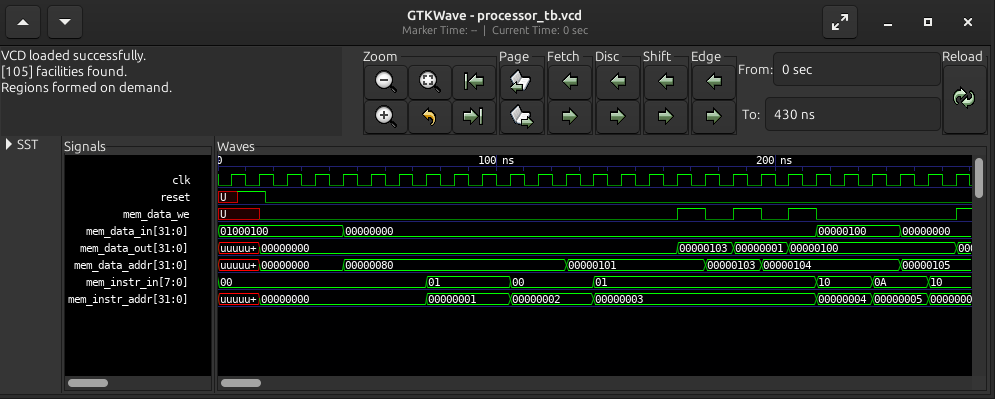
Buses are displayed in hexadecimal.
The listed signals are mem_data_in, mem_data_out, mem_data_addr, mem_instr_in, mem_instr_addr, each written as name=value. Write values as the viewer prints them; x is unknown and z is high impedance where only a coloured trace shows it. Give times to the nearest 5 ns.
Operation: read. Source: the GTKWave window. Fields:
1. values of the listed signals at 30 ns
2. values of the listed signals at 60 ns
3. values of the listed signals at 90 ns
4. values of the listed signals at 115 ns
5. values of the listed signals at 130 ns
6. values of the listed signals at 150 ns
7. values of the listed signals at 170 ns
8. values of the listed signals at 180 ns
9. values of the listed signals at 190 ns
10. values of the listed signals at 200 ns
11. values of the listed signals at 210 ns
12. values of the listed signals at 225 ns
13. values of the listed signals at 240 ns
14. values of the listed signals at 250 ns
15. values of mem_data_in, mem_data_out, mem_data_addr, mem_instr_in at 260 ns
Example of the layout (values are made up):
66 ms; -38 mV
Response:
mem_data_in=01000100, mem_data_out=00000000, mem_data_addr=00000000, mem_instr_in=00, mem_instr_addr=00000000; mem_data_in=00000000, mem_data_out=00000000, mem_data_addr=00000080, mem_instr_in=00, mem_instr_addr=00000000; mem_data_in=00000000, mem_data_out=00000000, mem_data_addr=00000080, mem_instr_in=01, mem_instr_addr=00000001; mem_data_in=00000000, mem_data_out=00000000, mem_data_addr=00000080, mem_instr_in=00, mem_instr_addr=00000002; mem_data_in=00000000, mem_data_out=00000000, mem_data_addr=00000101, mem_instr_in=00, mem_instr_addr=00000002; mem_data_in=00000000, mem_data_out=00000000, mem_data_addr=00000101, mem_instr_in=01, mem_instr_addr=00000003; mem_data_in=00000000, mem_data_out=00000103, mem_data_addr=00000101, mem_instr_in=01, mem_instr_addr=00000003; mem_data_in=00000000, mem_data_out=00000103, mem_data_addr=00000103, mem_instr_in=01, mem_instr_addr=00000003; mem_data_in=00000000, mem_data_out=00000001, mem_data_addr=00000103, mem_instr_in=01, mem_instr_addr=00000003; mem_data_in=00000000, mem_data_out=00000001, mem_data_addr=00000104, mem_instr_in=01, mem_instr_addr=00000003; mem_data_in=00000000, mem_data_out=00000100, mem_data_addr=00000104, mem_instr_in=01, mem_instr_addr=00000003; mem_data_in=00000100, mem_data_out=00000100, mem_data_addr=00000104, mem_instr_in=10, mem_instr_addr=00000004; mem_data_in=00000100, mem_data_out=00000100, mem_data_addr=00000104, mem_instr_in=0A, mem_instr_addr=00000005; mem_data_in=00000000, mem_data_out=00000100, mem_data_addr=00000105, mem_instr_in=0A, mem_instr_addr=00000005; mem_data_in=00000000, mem_data_out=00000100, mem_data_addr=00000105, mem_instr_in=10
